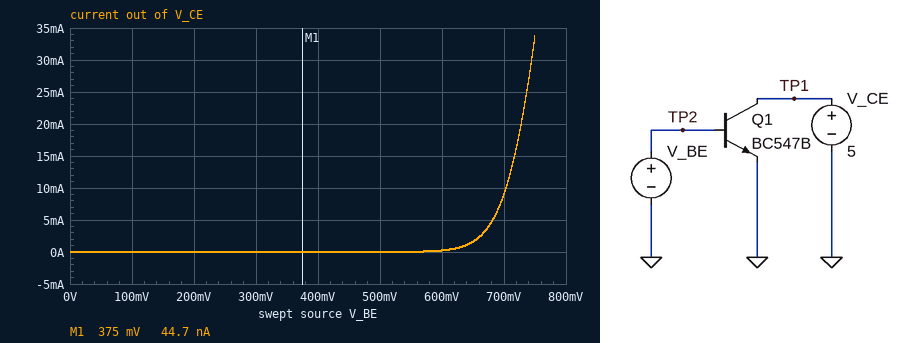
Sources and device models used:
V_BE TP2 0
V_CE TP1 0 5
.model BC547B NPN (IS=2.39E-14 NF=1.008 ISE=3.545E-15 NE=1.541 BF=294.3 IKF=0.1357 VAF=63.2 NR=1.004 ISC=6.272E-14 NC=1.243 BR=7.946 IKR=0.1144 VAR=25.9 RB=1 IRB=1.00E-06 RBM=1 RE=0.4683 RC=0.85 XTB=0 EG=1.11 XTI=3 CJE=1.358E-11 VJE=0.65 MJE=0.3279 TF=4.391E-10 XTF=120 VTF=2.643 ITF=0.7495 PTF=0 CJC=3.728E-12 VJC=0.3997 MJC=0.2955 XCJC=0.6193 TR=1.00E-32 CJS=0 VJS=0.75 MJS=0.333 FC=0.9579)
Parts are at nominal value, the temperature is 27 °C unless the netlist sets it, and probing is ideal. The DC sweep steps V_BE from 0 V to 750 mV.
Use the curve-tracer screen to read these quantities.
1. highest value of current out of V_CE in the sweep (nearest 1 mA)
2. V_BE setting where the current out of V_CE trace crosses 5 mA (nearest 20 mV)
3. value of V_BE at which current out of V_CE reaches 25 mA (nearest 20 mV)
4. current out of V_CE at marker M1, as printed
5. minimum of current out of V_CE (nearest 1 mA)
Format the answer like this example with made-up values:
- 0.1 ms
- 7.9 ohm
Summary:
- 34 mA
- 680 mV
- 740 mV
- 44.7 nA
- 0 A
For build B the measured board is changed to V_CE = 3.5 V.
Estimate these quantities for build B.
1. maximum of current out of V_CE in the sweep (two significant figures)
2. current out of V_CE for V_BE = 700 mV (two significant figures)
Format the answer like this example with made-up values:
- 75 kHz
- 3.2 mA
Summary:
- 33 mA
- 8.9 mA
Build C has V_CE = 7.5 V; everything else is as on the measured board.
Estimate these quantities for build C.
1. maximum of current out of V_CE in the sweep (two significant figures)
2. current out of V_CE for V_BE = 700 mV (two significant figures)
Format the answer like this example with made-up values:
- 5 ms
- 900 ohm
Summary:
- 35 mA
- 9.4 mA
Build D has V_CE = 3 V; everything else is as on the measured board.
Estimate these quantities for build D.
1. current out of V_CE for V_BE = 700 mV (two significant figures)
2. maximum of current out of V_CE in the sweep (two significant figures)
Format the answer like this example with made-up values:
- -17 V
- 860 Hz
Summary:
- 8.8 mA
- 33 mA
